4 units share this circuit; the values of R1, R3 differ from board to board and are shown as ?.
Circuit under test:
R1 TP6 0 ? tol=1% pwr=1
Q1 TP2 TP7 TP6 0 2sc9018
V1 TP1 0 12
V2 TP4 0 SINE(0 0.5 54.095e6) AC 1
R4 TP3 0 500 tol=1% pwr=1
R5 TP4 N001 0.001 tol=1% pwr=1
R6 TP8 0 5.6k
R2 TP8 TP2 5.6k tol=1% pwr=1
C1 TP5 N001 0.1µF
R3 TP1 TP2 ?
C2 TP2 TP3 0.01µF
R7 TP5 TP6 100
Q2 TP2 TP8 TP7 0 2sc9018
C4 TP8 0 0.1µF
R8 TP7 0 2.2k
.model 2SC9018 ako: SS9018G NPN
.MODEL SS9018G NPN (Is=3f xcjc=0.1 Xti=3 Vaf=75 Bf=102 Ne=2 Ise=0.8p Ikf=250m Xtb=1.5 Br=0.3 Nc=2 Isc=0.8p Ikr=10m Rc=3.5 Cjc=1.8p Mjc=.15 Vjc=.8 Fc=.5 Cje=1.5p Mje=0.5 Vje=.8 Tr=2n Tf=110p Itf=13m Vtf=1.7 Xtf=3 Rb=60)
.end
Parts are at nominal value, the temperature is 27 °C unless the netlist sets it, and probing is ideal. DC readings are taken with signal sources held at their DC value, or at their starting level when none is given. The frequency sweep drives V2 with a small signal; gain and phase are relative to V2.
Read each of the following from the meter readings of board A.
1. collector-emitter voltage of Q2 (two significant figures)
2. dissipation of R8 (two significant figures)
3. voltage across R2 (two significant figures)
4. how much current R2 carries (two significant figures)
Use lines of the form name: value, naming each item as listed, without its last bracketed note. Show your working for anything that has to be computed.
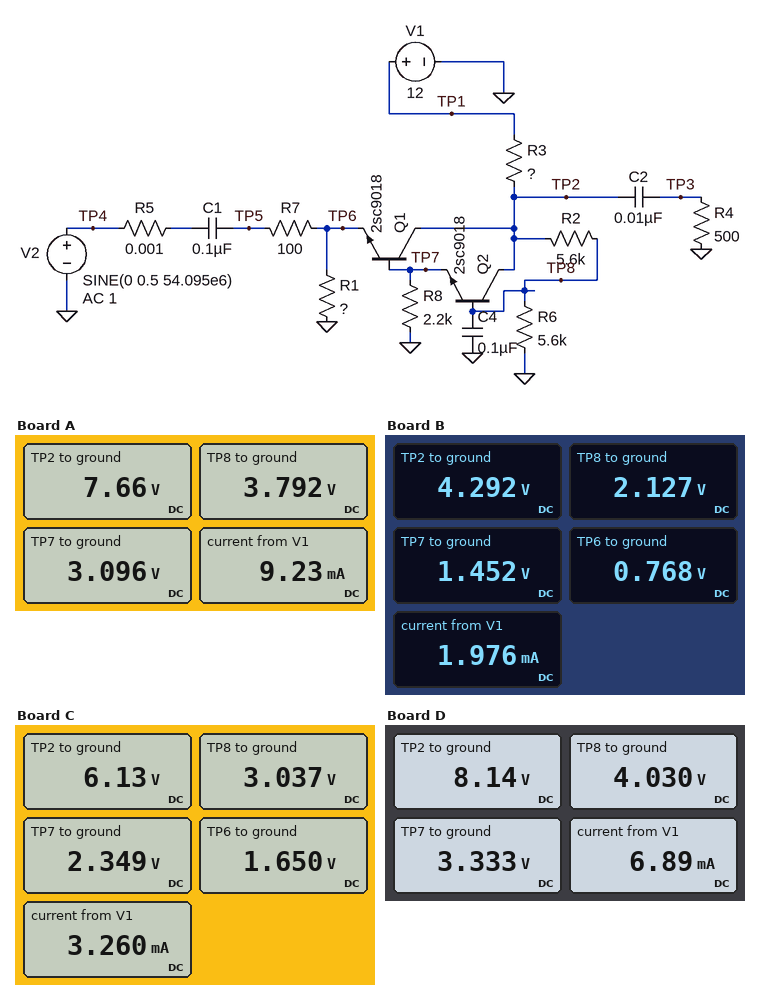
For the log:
collector-emitter voltage of Q2: 7.66 V - 3.096 V = 4.6 V
dissipation of R8: (3.096 V)^2 / 2.2 kΩ = 4.4 mW
voltage across R2: 7.66 V - 3.792 V = 3.9 V
how much current R2 carries: (7.66 V - 3.792 V) / 5.6 kΩ = 690 µA
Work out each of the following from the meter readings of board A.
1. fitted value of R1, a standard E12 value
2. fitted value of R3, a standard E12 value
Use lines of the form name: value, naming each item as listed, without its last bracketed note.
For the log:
fitted value of R1, a standard E12 value: 330 Ω
fitted value of R3, a standard E12 value: 470 Ω
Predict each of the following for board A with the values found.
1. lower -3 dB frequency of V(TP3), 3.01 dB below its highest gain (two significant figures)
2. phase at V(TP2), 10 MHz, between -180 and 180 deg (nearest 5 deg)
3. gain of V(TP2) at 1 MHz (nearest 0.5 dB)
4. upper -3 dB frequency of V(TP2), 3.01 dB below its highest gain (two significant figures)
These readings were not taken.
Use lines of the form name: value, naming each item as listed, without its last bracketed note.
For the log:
lower -3 dB frequency of V(TP3), 3.01 dB below its highest gain: 25 kHz
phase at V(TP2), 10 MHz, between -180 and 180 deg: 0 deg
gain of V(TP2) at 1 MHz: 7.0 dB
upper -3 dB frequency of V(TP2), 3.01 dB below its highest gain: 280 MHz
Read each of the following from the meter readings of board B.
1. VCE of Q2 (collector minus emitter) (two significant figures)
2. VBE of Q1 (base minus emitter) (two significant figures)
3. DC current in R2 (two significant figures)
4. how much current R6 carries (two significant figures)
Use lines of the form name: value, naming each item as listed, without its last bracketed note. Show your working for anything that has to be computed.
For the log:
VCE of Q2 (collector minus emitter): 4.292 V - 1.452 V = 2.8 V
VBE of Q1 (base minus emitter): 1.452 V - 768 mV = 680 mV
DC current in R2: (4.292 V - 2.127 V) / 5.6 kΩ = 390 µA
how much current R6 carries: (2.127 V) / 5.6 kΩ = 380 µA
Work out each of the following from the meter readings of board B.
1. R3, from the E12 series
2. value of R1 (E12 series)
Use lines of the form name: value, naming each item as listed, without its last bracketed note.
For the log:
R3, from the E12 series: 3.9 kΩ
value of R1: 820 Ω
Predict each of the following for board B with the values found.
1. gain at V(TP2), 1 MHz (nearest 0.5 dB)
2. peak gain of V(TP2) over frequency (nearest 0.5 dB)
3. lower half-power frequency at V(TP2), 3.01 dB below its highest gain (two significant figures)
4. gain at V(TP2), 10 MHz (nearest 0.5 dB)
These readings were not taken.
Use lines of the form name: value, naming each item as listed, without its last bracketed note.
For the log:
gain at V(TP2), 1 MHz: 10.0 dB
peak gain of V(TP2) over frequency: 15.0 dB
lower half-power frequency at V(TP2), 3.01 dB below its highest gain: 4.5 kHz
gain at V(TP2), 10 MHz: 10.0 dB
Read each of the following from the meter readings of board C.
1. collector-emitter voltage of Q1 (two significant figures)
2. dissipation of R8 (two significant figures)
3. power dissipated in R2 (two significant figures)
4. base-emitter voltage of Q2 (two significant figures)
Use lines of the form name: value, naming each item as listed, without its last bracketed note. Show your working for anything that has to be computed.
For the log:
collector-emitter voltage of Q1: 6.13 V - 1.65 V = 4.5 V
dissipation of R8: (2.349 V)^2 / 2.2 kΩ = 2.5 mW
power dissipated in R2: (6.13 V - 3.037 V)^2 / 5.6 kΩ = 1.7 mW
base-emitter voltage of Q2: 3.037 V - 2.349 V = 690 mV
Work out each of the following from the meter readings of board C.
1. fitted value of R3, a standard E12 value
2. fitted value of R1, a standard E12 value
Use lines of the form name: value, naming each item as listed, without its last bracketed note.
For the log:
fitted value of R3, a standard E12 value: 1.8 kΩ
fitted value of R1, a standard E12 value: 1 kΩ
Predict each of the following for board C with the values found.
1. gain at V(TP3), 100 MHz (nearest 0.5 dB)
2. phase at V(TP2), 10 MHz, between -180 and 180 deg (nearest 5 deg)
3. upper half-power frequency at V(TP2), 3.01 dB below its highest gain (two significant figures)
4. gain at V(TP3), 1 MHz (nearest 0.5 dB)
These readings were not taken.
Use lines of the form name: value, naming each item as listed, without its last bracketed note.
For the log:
gain at V(TP3), 100 MHz: 9.5 dB
phase at V(TP2), 10 MHz, between -180 and 180 deg: -5 deg
upper half-power frequency at V(TP2), 3.01 dB below its highest gain: 80 kHz
gain at V(TP3), 1 MHz: 10.0 dB
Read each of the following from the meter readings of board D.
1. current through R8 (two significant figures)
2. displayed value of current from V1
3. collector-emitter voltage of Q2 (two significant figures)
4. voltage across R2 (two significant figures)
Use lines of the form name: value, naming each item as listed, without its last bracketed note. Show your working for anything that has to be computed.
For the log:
current through R8: (3.333 V) / 2.2 kΩ = 1.5 mA
displayed value of current from V1: 6.89 mA
collector-emitter voltage of Q2: 8.14 V - 3.333 V = 4.8 V
voltage across R2: 8.14 V - 4.03 V = 4.1 V
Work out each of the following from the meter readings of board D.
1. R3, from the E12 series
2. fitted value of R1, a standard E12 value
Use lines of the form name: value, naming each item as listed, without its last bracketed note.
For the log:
R3, from the E12 series: 560 Ω
fitted value of R1, a standard E12 value: 560 Ω
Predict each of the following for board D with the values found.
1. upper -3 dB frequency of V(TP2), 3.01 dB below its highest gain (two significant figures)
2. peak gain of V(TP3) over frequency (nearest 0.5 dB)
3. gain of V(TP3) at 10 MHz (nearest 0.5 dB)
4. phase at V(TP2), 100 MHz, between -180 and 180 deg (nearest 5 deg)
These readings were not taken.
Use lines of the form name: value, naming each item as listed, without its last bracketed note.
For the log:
upper -3 dB frequency of V(TP2), 3.01 dB below its highest gain: 270 MHz
peak gain of V(TP3) over frequency: 7.5 dB
gain of V(TP3) at 10 MHz: 7.5 dB
phase at V(TP2), 100 MHz, between -180 and 180 deg: -20 deg
